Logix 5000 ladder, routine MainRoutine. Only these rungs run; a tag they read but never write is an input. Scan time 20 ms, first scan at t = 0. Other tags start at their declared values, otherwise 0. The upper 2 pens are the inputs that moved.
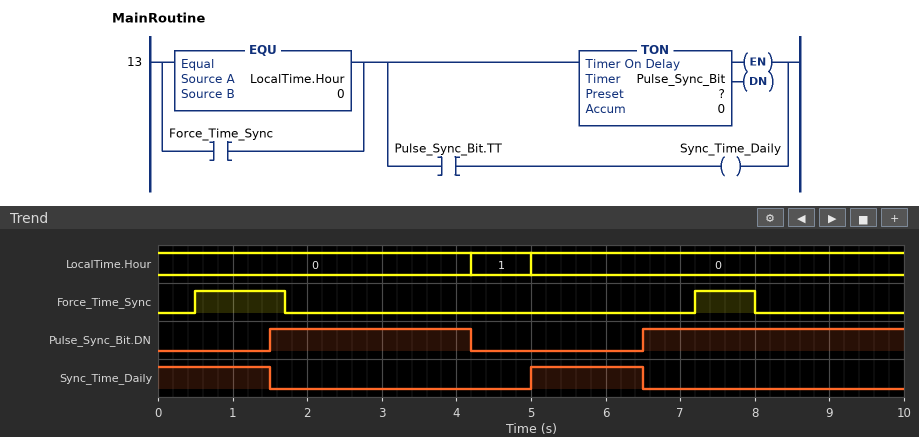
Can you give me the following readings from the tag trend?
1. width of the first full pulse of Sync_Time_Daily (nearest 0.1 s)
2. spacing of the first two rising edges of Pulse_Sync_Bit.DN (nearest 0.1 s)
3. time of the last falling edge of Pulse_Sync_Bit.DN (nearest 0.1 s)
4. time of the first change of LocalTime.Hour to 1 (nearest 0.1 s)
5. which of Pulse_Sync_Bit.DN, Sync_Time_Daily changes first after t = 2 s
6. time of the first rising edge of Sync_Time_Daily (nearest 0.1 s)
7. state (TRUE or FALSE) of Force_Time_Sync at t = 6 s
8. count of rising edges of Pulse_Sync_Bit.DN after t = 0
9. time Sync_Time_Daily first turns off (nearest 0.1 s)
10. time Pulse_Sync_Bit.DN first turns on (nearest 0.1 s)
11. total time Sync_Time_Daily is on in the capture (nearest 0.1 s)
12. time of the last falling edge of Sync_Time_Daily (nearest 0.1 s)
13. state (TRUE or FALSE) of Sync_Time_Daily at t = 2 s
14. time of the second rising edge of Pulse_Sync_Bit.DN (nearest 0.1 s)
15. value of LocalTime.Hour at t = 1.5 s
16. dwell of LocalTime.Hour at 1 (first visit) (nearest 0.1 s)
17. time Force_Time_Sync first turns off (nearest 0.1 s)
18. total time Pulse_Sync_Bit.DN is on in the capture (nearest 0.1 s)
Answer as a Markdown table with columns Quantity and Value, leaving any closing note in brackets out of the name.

| Quantity | Value |
|---|---|
| width of the first full pulse of Sync_Time_Daily | 1.5 s |
| spacing of the first two rising edges of Pulse_Sync_Bit.DN | 5.0 s |
| time of the last falling edge of Pulse_Sync_Bit.DN | 4.2 s |
| time of the first change of LocalTime.Hour to 1 | 4.2 s |
| which of Pulse_Sync_Bit.DN, Sync_Time_Daily changes first after t = 2 s | Pulse_Sync_Bit.DN |
| time of the first rising edge of Sync_Time_Daily | 5.0 s |
| state (TRUE or FALSE) of Force_Time_Sync at t = 6 s | FALSE |
| count of rising edges of Pulse_Sync_Bit.DN after t = 0 | 2 |
| time Sync_Time_Daily first turns off | 1.5 s |
| time Pulse_Sync_Bit.DN first turns on | 1.5 s |
| total time Sync_Time_Daily is on in the capture | 3.0 s |
| time of the last falling edge of Sync_Time_Daily | 6.5 s |
| state (TRUE or FALSE) of Sync_Time_Daily at t = 2 s | FALSE |
| time of the second rising edge of Pulse_Sync_Bit.DN | 6.5 s |
| value of LocalTime.Hour at t = 1.5 s | 0 |
| dwell of LocalTime.Hour at 1 (first visit) | 0.8 s |
| time Force_Time_Sync first turns off | 1.7 s |
| total time Pulse_Sync_Bit.DN is on in the capture | 6.2 s |
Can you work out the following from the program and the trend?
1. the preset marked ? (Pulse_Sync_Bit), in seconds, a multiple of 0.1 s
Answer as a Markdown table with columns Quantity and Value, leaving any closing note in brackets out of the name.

| Quantity | Value |
|---|---|
| the preset marked ? (Pulse_Sync_Bit), in seconds, a multiple of 0.1 s | 1.5 s |
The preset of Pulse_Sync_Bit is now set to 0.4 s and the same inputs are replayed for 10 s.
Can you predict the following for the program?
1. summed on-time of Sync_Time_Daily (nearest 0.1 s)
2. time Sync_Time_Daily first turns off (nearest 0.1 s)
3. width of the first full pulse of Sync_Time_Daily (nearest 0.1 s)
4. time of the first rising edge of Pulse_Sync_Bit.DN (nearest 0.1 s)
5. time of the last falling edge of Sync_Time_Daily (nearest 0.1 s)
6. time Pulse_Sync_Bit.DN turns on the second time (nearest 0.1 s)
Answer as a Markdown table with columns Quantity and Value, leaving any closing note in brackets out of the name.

| Quantity | Value |
|---|---|
| summed on-time of Sync_Time_Daily | 0.8 s |
| time Sync_Time_Daily first turns off | 0.4 s |
| width of the first full pulse of Sync_Time_Daily | 0.4 s |
| time of the first rising edge of Pulse_Sync_Bit.DN | 0.4 s |
| time of the last falling edge of Sync_Time_Daily | 5.4 s |
| time Pulse_Sync_Bit.DN turns on the second time | 5.4 s |
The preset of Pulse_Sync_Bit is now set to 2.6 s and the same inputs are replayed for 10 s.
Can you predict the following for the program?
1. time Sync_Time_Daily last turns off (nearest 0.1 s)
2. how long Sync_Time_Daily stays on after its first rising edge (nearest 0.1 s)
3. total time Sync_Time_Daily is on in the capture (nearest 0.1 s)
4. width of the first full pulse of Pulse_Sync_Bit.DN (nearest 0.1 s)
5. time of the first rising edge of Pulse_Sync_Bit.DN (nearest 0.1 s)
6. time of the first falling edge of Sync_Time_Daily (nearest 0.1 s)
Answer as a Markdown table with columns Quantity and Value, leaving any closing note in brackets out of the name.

| Quantity | Value |
|---|---|
| time Sync_Time_Daily last turns off | 7.6 s |
| how long Sync_Time_Daily stays on after its first rising edge | 2.6 s |
| total time Sync_Time_Daily is on in the capture | 5.2 s |
| width of the first full pulse of Pulse_Sync_Bit.DN | 1.6 s |
| time of the first rising edge of Pulse_Sync_Bit.DN | 2.6 s |
| time of the first falling edge of Sync_Time_Daily | 2.6 s |
